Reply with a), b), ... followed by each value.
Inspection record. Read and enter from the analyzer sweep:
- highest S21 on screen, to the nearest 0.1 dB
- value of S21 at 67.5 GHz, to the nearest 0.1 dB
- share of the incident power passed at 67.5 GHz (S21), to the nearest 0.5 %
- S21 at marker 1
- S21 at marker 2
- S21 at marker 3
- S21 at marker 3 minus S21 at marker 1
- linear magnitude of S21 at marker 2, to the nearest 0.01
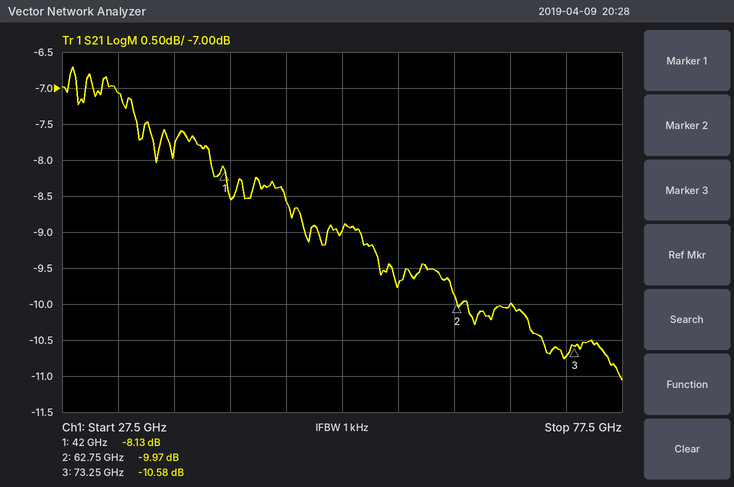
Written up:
a) -6.7 dB
b) -10.0 dB
c) 10.0 %
d) -8.13 dB
e) -9.97 dB
f) -10.58 dB
g) -2.45 dB
h) 0.32
